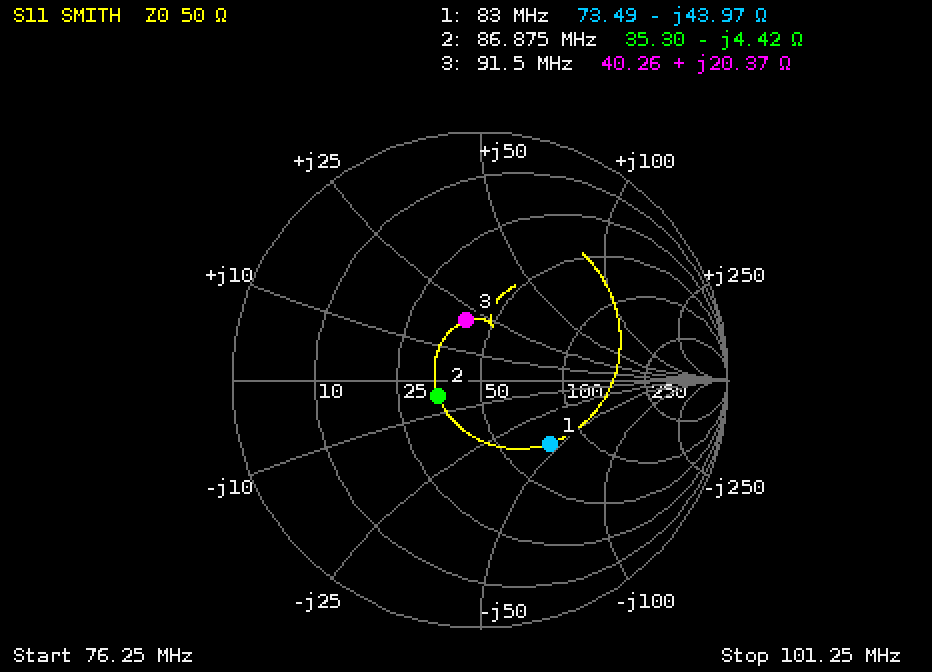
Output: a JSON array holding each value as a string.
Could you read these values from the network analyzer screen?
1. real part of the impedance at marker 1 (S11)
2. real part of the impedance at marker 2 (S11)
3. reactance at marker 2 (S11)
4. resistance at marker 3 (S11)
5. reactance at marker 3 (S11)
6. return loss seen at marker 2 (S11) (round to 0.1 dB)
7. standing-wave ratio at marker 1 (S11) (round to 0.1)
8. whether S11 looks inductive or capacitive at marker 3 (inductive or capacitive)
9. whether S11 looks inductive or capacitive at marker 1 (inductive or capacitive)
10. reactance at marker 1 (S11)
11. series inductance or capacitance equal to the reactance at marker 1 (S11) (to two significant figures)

["73.49 Ω", "35.30 Ω", "-4.42 Ω", "40.26 Ω", "+20.37 Ω", "14.9 dB", "2.2", "inductive", "capacitive", "-43.97 Ω", "44 pF"]
